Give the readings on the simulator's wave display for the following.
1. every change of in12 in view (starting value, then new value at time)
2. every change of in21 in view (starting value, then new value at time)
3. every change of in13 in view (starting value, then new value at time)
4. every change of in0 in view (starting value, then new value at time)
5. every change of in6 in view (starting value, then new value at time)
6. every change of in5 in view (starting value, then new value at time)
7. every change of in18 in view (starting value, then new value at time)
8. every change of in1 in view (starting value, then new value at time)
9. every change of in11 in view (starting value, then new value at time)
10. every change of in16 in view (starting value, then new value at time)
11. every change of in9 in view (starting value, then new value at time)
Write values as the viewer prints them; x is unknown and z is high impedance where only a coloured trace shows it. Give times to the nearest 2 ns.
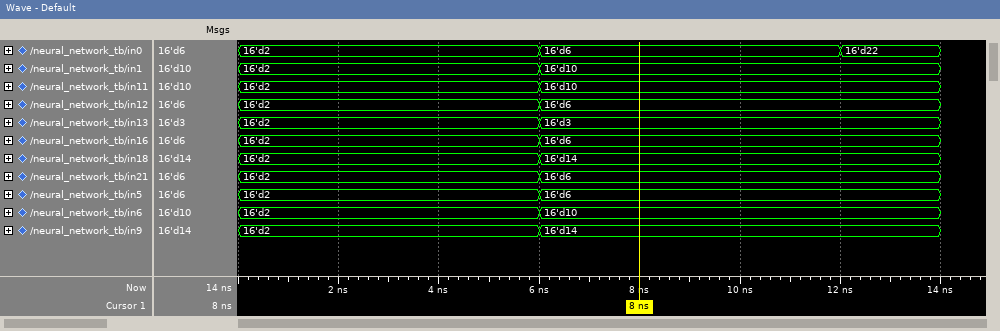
16'd2, 16'd6 at 6 ns
16'd2, 16'd6 at 6 ns
16'd2, 16'd3 at 6 ns
16'd2, 16'd6 at 6 ns, 16'd22 at 12 ns
16'd2, 16'd10 at 6 ns
16'd2, 16'd6 at 6 ns
16'd2, 16'd14 at 6 ns
16'd2, 16'd10 at 6 ns
16'd2, 16'd10 at 6 ns
16'd2, 16'd6 at 6 ns
16'd2, 16'd14 at 6 ns
